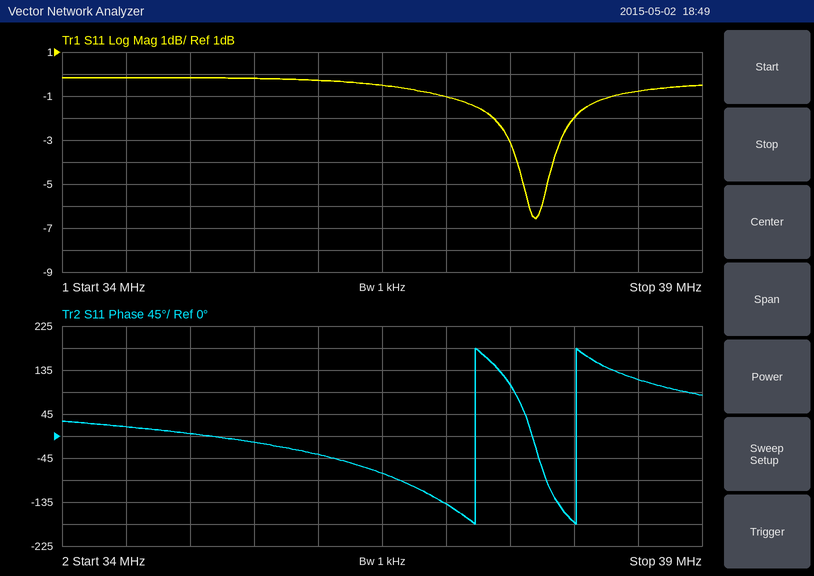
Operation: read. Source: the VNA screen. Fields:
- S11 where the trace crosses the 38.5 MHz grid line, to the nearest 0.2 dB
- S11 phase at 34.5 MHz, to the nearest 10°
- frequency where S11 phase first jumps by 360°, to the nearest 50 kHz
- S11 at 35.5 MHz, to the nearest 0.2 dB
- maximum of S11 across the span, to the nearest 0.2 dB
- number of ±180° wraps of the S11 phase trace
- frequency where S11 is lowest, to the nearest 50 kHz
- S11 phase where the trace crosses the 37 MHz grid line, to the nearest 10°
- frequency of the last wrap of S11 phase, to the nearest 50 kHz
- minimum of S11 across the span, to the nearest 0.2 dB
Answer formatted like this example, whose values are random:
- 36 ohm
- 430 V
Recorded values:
- -0.8 dB
- 20°
- 37.25 MHz
- -0.2 dB
- -0.2 dB
- 2
- 37.70 MHz
- -140°
- 38.00 MHz
- -6.6 dB
